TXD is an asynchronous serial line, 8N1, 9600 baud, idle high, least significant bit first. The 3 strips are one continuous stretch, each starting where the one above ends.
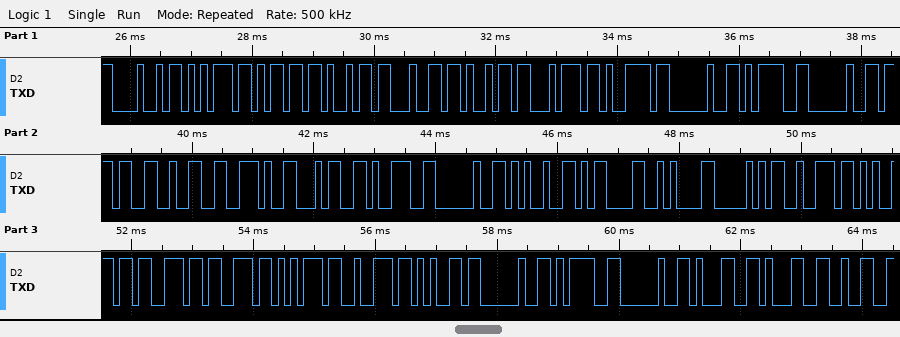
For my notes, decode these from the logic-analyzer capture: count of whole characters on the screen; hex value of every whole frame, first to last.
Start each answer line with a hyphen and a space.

- 34
- 48 75 6D 69 64 69 74 79 20 3D 20 37 32 2E 34 39 20 25 0D 0A 50 72 65 73 73 75 72 65 20 3D 20 31 31 32
